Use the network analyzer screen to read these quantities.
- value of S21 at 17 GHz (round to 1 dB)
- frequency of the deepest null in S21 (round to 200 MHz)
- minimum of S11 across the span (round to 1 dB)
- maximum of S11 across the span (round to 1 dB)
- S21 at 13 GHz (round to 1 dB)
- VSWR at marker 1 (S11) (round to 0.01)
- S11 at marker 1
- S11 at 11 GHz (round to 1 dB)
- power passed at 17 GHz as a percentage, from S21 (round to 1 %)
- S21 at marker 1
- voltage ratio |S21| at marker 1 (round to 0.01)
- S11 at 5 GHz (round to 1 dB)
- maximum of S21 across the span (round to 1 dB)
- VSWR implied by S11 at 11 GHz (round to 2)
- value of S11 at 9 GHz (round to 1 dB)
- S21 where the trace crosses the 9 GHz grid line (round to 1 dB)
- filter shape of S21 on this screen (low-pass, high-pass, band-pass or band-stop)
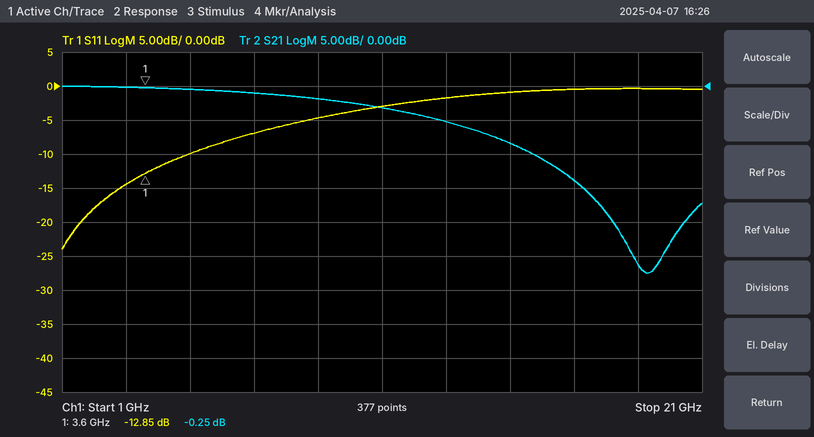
-14 dB
19.2 GHz
-24 dB
0 dB
-5 dB
1.59
-12.85 dB
-3 dB
4 %
-0.25 dB
0.97
-10 dB
0 dB
6
-5 dB
-2 dB
low-pass
